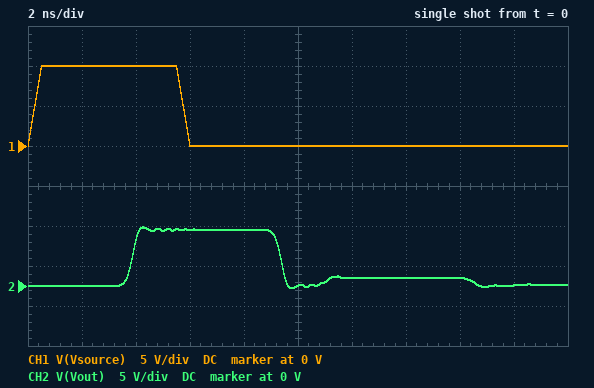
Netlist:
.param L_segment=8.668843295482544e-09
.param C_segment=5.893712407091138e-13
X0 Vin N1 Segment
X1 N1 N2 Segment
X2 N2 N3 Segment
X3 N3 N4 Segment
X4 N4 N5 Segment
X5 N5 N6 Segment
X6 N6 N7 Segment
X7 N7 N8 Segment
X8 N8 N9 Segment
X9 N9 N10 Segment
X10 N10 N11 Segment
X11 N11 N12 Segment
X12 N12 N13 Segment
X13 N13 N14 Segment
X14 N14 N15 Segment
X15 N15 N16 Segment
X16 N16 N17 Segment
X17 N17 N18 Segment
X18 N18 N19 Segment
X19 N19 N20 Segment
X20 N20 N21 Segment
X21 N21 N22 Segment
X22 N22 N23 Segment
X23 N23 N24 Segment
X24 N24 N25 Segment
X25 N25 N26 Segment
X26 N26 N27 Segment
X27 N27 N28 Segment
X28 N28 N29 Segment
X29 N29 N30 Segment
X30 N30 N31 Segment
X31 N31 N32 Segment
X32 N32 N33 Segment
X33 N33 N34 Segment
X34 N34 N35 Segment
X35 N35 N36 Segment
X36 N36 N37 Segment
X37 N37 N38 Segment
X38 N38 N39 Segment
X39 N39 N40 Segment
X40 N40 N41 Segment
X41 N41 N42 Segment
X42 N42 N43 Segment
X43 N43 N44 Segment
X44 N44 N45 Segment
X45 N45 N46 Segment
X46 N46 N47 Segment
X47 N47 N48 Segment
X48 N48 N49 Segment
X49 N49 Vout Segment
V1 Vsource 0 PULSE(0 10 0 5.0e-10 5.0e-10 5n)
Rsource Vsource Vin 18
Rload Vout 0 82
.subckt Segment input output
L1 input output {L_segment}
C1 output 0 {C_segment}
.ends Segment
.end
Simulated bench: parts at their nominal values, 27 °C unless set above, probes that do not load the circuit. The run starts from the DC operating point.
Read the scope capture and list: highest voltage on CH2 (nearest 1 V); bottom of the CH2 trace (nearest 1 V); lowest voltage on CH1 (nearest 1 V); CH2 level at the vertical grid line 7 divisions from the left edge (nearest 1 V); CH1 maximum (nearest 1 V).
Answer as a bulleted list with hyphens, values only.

- 7 V
- 0 V
- 0 V
- 1 V
- 10 V
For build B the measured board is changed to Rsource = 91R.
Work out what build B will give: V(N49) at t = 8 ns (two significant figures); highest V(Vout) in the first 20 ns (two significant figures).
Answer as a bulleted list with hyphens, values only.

- 4.6 V
- 4.8 V
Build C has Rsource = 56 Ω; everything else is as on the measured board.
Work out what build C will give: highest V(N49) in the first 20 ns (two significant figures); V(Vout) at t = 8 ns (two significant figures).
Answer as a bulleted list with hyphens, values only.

- 5.7 V
- 5.5 V
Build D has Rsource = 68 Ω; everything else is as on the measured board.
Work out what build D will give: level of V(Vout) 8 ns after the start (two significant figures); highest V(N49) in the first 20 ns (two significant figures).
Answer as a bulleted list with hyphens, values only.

- 5.2 V
- 5.4 V
